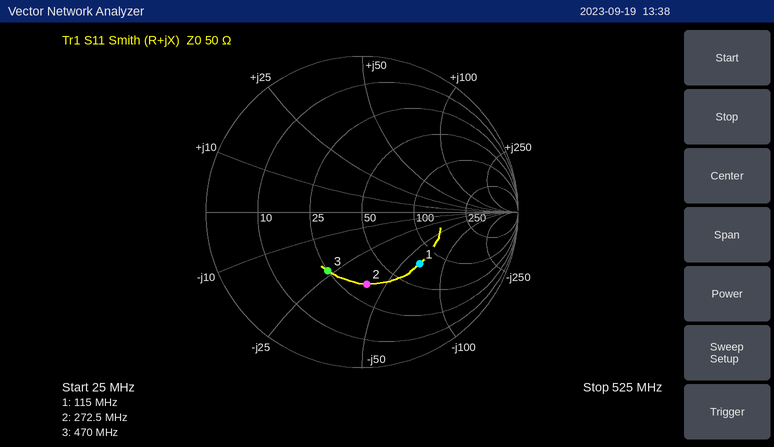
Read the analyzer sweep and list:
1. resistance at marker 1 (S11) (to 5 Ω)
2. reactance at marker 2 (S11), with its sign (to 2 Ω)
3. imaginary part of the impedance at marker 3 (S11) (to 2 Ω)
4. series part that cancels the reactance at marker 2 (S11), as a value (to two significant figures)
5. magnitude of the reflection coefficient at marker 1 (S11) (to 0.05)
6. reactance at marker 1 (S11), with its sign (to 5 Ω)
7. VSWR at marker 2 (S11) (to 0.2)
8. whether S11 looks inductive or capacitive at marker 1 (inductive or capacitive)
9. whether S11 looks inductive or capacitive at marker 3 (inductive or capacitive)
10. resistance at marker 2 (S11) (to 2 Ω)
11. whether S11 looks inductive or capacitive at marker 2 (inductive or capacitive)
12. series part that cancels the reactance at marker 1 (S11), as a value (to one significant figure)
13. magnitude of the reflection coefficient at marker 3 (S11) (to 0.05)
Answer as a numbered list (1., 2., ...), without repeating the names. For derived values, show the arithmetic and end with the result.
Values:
1. 75 Ω
2. -40 Ω
3. -24 Ω
4. L = 40 Ω/(2π × 272.5 MHz) ≈ 23 nH
5. 0.50
6. -65 Ω
7. 2.8
8. capacitive
9. capacitive
10. 34 Ω
11. capacitive
12. L = 65 Ω/(2π × 115 MHz) ≈ 90 nH
13. 0.45
